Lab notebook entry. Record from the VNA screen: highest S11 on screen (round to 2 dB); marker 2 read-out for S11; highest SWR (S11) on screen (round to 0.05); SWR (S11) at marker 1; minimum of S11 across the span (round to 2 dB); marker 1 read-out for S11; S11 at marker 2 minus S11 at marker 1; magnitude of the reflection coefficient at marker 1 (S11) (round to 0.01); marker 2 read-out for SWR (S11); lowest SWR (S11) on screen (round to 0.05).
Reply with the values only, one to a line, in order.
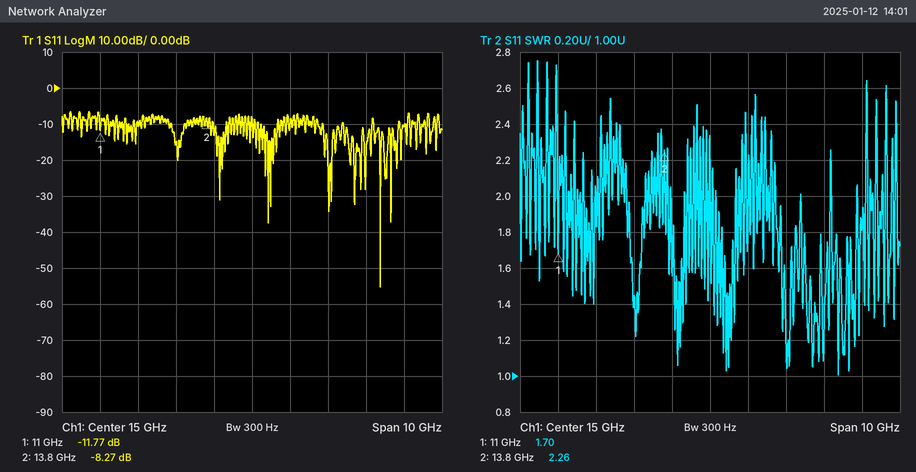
-6 dB
-8.27 dB
2.75
1.70
-56 dB
-11.77 dB
3.50 dB
0.26
2.26
1.00
